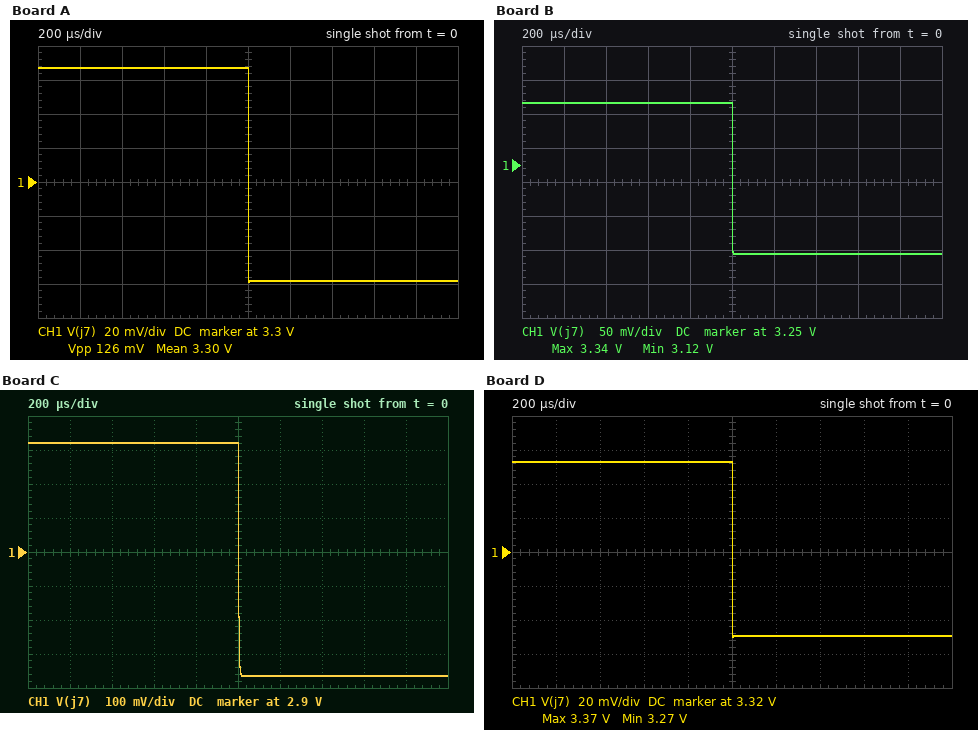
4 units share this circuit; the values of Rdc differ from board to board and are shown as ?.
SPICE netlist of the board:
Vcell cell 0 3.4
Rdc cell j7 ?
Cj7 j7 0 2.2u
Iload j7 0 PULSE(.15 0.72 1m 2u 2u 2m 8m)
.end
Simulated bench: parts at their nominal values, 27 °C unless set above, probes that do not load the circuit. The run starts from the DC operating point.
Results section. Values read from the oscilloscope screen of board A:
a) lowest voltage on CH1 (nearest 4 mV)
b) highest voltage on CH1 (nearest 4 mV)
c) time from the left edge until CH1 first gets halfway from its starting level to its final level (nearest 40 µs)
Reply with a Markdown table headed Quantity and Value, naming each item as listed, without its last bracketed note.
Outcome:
| Quantity | Value |
|---|---|
| lowest voltage on CH1 | 3.240 V |
| highest voltage on CH1 | 3.368 V |
| time from the left edge until CH1 first gets halfway from its starting level to its final level | 1.00 ms |
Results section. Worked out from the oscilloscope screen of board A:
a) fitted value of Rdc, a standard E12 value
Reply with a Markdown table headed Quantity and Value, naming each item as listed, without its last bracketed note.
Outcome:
| Quantity | Value |
|---|---|
| fitted value of Rdc, a standard E12 value | 0.22 Ω |
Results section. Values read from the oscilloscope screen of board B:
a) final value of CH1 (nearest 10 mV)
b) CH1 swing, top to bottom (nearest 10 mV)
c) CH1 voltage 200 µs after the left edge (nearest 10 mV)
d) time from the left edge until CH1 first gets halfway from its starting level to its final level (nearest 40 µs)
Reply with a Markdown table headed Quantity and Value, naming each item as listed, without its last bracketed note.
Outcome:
| Quantity | Value |
|---|---|
| final value of CH1 | 3.12 V |
| CH1 swing, top to bottom | 220 mV |
| CH1 voltage 200 µs after the left edge | 3.34 V |
| time from the left edge until CH1 first gets halfway from its starting level to its final level | 1.00 ms |
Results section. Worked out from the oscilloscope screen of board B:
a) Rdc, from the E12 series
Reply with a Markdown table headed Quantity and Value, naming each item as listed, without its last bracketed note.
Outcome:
| Quantity | Value |
|---|---|
| Rdc, from the E12 series | 0.39 Ω |
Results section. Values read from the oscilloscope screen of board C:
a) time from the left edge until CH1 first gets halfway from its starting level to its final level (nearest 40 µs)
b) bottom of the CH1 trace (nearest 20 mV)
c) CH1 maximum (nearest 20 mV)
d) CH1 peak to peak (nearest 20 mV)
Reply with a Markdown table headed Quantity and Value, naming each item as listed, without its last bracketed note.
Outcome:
| Quantity | Value |
|---|---|
| time from the left edge until CH1 first gets halfway from its starting level to its final level | 1.00 ms |
| bottom of the CH1 trace | 2.54 V |
| CH1 maximum | 3.22 V |
| CH1 peak to peak | 680 mV |
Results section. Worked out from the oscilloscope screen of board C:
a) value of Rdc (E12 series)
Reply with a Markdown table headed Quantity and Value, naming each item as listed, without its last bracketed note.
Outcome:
| Quantity | Value |
|---|---|
| value of Rdc | 1.2 Ω |
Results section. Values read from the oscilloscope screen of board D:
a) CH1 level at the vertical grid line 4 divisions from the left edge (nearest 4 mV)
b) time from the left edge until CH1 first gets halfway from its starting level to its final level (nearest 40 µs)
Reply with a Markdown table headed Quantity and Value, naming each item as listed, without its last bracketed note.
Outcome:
| Quantity | Value |
|---|---|
| CH1 level at the vertical grid line 4 divisions from the left edge | 3.372 V |
| time from the left edge until CH1 first gets halfway from its starting level to its final level | 1.00 ms |
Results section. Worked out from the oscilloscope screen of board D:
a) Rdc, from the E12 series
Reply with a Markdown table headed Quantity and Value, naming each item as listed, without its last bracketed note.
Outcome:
| Quantity | Value |
|---|---|
| Rdc, from the E12 series | 0.18 Ω |
